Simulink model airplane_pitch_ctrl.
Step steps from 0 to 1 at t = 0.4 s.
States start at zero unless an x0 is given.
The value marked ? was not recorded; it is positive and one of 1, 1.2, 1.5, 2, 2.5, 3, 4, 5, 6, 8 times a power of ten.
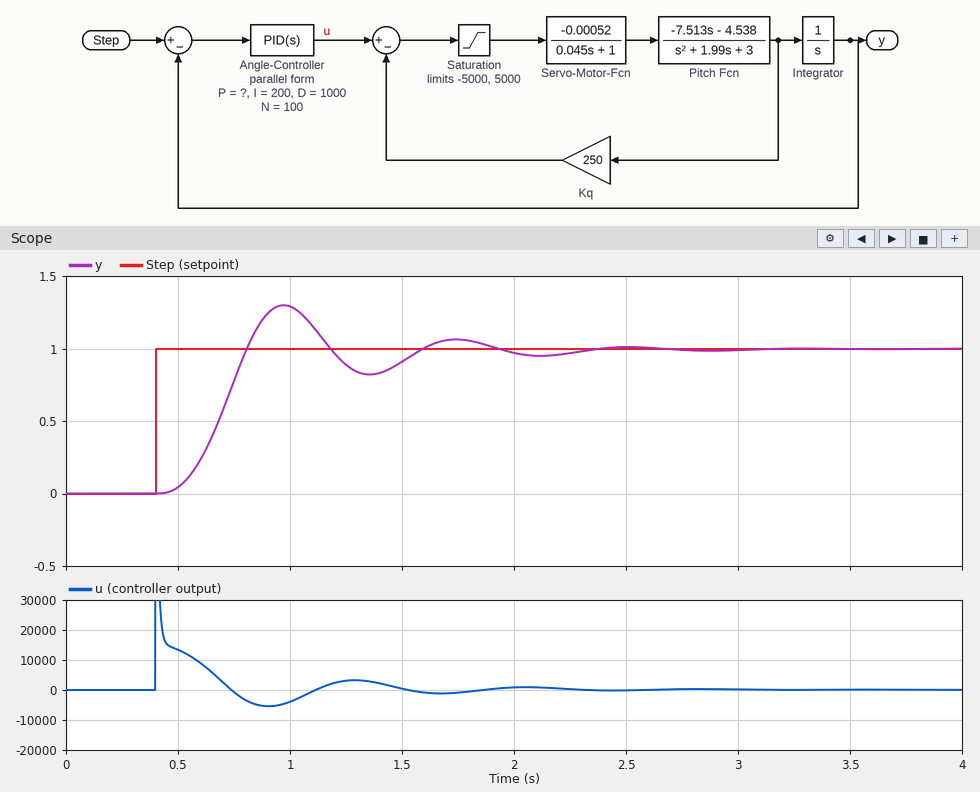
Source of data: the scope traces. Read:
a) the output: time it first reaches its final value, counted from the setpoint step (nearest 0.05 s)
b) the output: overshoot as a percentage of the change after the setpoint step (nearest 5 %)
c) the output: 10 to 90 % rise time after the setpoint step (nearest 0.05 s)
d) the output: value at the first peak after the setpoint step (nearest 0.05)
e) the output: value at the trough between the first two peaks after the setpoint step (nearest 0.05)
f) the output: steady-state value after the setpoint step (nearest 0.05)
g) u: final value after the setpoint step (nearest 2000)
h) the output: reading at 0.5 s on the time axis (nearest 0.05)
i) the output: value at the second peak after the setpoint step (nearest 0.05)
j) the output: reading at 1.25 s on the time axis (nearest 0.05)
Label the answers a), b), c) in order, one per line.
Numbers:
a) 0.40 s
b) 30 %
c) 0.25 s
d) 1.30
e) 0.80
f) 1.00
g) 0
h) 0.05
i) 1.05
j) 0.90
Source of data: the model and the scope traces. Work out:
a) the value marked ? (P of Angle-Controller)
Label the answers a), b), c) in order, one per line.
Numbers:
a) 15000
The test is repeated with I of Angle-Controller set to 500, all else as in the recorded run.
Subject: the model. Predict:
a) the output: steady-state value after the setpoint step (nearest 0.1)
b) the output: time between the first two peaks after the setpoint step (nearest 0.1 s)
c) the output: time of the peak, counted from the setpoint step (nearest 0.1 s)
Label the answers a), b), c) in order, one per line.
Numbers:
a) 1.0
b) 0.8 s
c) 0.6 s
